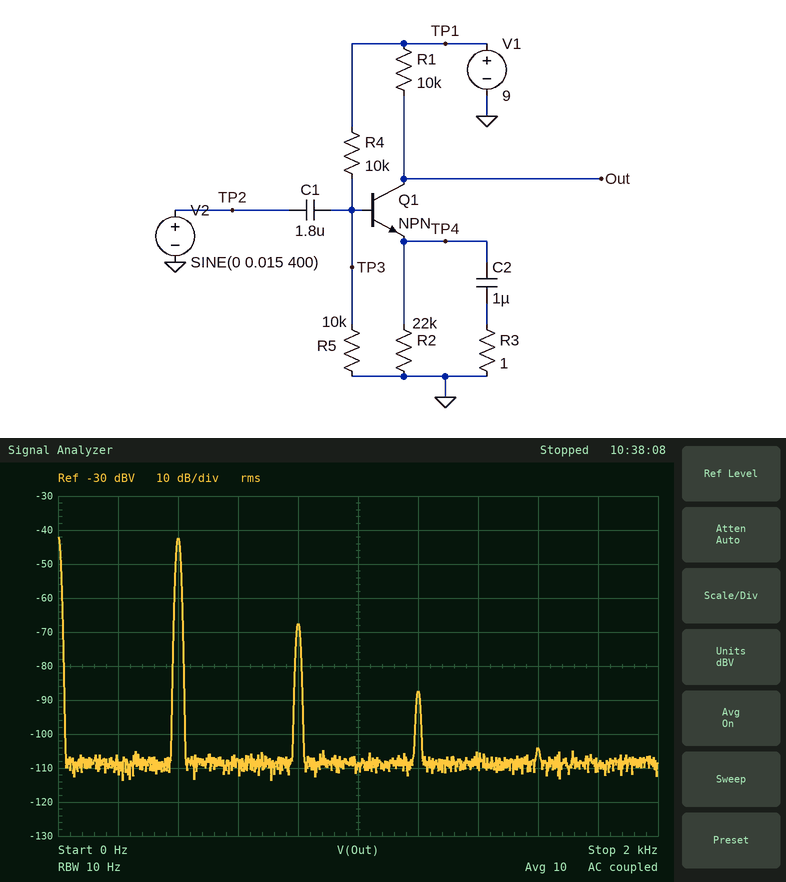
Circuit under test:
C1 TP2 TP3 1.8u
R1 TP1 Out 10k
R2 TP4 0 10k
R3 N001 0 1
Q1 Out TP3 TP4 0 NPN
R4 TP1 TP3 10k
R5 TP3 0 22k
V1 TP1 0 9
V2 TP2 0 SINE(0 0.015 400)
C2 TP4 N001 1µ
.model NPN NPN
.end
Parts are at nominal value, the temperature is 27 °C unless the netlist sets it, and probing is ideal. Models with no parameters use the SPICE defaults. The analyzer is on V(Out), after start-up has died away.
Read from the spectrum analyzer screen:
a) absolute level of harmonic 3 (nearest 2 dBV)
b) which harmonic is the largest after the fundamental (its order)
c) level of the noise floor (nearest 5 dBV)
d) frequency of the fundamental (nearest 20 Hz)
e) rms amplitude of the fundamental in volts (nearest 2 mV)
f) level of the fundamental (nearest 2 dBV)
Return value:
-88 dBV
2
-110 dBV
400 Hz
8 mV
-42 dBV
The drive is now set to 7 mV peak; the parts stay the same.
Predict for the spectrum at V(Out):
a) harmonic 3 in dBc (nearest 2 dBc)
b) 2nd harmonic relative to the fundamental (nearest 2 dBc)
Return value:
-58 dBc
-32 dBc
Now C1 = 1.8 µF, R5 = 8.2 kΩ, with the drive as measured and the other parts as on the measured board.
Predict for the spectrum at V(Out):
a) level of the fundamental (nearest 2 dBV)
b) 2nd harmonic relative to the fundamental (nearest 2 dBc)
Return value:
-12 dBV
-40 dBc
